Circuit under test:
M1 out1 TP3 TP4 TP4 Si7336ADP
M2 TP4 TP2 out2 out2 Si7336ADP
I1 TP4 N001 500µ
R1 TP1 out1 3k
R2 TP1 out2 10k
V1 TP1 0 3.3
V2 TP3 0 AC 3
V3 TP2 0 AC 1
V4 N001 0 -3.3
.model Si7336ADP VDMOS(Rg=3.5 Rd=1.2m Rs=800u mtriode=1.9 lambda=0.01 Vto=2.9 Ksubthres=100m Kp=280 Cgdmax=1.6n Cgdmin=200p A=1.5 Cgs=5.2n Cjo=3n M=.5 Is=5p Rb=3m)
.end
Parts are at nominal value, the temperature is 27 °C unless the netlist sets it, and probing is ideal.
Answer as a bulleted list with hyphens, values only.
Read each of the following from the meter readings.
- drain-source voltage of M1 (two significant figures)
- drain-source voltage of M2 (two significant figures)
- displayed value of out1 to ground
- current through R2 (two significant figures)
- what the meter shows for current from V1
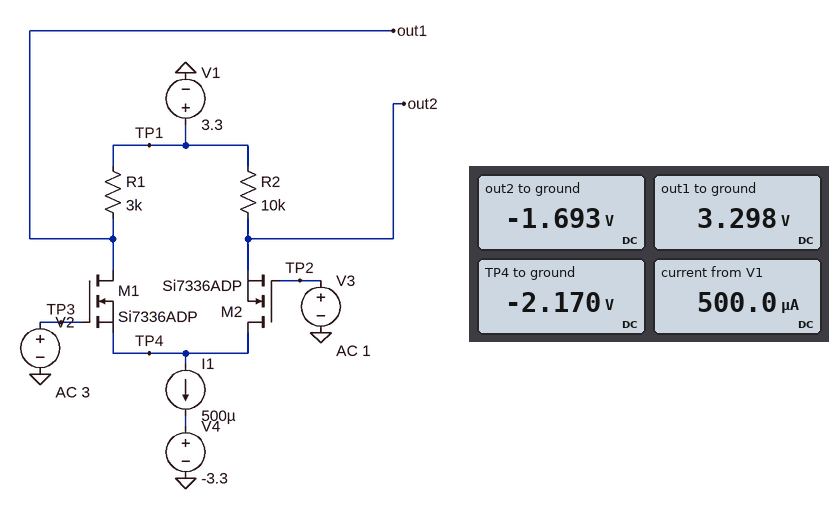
- 5.5 V
- -480 mV
- 3.298 V
- 500 µA
- 500.0 µA
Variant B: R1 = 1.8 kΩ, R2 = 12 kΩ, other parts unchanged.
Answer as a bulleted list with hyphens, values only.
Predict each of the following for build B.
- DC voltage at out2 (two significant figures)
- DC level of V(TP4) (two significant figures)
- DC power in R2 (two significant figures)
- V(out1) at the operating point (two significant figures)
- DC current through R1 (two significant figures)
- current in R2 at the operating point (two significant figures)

- -1.9 V
- -2.4 V
- 2.3 mW
- 3.2 V
- 64 µA
- 440 µA
